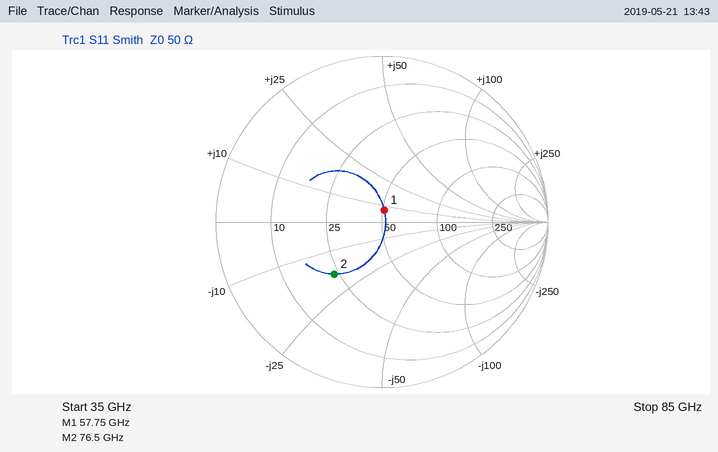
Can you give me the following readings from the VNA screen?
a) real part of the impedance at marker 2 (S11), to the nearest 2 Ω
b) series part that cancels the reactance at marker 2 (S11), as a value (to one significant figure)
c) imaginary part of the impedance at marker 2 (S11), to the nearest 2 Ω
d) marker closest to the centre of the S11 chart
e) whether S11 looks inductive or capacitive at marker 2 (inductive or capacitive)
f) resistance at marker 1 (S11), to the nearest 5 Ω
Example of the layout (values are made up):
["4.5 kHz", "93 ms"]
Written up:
["24 Ω", "40 pH", "-18 Ω", "marker 1", "capacitive", "50 Ω"]
